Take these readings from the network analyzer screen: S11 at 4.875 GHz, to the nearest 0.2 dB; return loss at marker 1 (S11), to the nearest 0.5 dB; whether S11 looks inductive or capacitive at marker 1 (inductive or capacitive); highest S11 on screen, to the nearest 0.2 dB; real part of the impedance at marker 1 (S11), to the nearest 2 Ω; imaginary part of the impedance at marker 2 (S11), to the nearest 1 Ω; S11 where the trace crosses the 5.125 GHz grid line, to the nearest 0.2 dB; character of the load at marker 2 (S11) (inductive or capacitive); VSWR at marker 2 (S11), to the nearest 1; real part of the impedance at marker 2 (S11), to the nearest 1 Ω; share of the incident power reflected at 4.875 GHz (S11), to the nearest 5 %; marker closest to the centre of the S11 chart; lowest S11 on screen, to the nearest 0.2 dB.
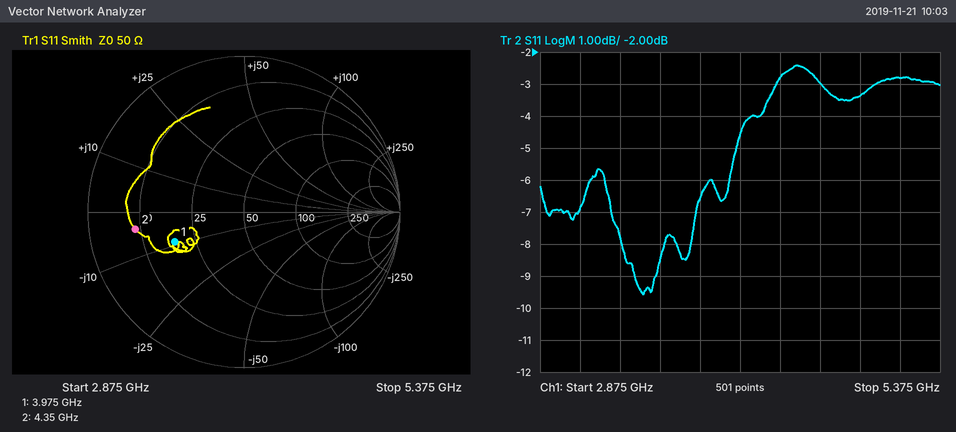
-3.4 dB
6.5 dB
capacitive
-2.4 dB
18 Ω
-4 Ω
-2.8 dB
capacitive
6
9 Ω
45 %
marker 1
-9.6 dB
